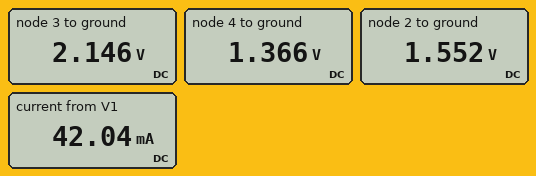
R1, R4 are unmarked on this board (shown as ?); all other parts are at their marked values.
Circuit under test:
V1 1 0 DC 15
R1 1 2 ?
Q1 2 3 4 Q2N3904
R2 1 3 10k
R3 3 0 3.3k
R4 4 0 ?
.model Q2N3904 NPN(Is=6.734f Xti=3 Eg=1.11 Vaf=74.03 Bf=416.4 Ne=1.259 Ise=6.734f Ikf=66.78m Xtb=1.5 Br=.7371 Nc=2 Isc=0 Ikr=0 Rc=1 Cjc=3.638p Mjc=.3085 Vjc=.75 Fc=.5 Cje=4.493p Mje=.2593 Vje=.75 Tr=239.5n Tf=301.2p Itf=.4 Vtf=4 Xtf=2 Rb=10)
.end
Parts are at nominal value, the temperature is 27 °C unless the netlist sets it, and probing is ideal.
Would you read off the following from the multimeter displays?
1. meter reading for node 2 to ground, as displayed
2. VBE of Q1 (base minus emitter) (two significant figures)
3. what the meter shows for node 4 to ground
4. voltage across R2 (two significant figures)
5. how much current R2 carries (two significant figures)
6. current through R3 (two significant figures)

1.552 V
780 mV
1.366 V
13 V
1.3 mA
650 µA
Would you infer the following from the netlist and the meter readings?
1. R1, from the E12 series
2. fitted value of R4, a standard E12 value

330 Ω
33 Ω
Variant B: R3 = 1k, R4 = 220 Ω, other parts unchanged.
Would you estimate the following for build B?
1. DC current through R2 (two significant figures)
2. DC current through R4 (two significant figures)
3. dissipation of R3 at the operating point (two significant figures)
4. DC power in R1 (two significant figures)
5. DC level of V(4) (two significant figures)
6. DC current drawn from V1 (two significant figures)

1.4 mA
3.0 mA
1.8 mW
2.9 mW
660 mV
4.3 mA
